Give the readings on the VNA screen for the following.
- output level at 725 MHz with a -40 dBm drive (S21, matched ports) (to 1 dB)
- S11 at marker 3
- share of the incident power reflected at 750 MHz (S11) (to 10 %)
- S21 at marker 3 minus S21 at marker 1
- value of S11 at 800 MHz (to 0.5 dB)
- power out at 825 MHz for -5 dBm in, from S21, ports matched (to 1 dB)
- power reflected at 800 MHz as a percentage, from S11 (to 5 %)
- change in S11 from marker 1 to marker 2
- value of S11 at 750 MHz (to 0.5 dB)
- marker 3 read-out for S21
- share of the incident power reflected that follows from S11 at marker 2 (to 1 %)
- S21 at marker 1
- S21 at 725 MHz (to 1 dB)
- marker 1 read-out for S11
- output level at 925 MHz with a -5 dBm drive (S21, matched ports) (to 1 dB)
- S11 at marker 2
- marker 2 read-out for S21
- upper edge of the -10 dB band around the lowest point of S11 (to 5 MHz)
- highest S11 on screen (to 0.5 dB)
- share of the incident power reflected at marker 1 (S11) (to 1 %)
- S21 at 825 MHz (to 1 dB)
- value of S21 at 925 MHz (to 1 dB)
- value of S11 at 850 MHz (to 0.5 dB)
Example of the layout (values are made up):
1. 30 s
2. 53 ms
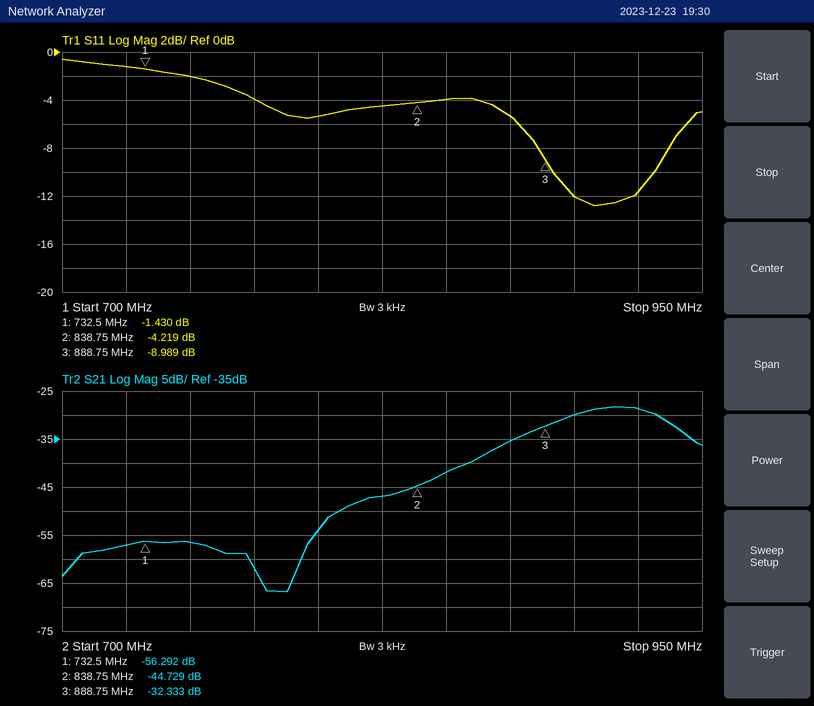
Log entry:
1. -97 dBm
2. -8.989 dB
3. 60 %
4. 23.959 dB
5. -5.5 dB
6. -52 dBm
7. 30 %
8. -2.789 dB
9. -2.0 dB
10. -32.333 dB
11. 38 %
12. -56.292 dB
13. -57 dB
14. -1.430 dB
15. -34 dBm
16. -4.219 dB
17. -44.729 dB
18. 930 MHz
19. -0.5 dB
20. 72 %
21. -47 dB
22. -29 dB
23. -4.0 dB
